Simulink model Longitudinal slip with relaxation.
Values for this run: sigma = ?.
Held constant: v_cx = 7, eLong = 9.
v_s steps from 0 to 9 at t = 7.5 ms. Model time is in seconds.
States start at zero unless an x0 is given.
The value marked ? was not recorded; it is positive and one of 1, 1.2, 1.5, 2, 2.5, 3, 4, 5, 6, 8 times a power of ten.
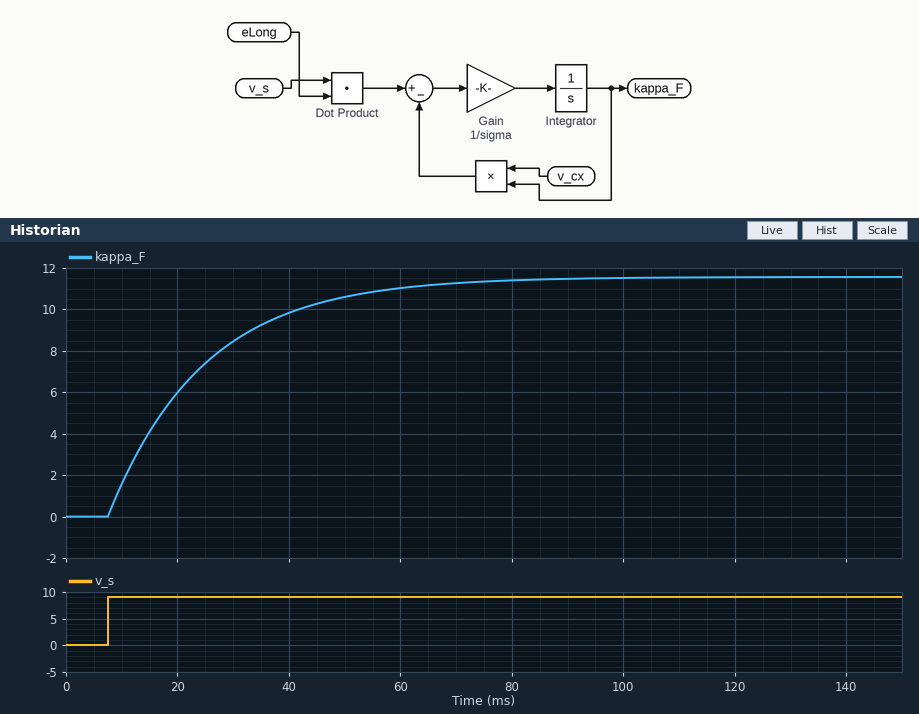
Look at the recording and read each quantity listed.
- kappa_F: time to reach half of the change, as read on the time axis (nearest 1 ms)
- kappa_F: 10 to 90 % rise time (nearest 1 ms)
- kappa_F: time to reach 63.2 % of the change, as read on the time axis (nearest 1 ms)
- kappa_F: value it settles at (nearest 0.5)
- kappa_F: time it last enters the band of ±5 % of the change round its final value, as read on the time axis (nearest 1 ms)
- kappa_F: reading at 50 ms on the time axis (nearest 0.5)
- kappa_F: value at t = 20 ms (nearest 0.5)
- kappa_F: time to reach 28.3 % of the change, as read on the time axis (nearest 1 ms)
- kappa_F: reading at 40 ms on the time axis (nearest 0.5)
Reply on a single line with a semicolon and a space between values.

19 ms; 38 ms; 25 ms; 11.5; 59 ms; 10.5; 6.0; 13 ms; 10.0
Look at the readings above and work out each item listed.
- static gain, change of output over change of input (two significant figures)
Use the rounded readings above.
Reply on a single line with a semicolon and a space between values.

1.3
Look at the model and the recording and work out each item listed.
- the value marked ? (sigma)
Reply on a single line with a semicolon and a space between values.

0.12
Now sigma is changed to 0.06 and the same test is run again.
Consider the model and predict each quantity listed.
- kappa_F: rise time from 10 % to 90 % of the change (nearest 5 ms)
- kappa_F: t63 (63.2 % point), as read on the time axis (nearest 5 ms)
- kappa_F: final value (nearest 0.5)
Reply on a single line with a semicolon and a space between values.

20 ms; 15 ms; 11.5
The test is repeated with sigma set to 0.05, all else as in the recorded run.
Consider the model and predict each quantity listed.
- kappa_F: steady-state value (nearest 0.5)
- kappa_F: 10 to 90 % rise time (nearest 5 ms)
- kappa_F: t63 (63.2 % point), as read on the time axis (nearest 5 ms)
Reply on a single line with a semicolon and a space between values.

11.5; 15 ms; 15 ms
